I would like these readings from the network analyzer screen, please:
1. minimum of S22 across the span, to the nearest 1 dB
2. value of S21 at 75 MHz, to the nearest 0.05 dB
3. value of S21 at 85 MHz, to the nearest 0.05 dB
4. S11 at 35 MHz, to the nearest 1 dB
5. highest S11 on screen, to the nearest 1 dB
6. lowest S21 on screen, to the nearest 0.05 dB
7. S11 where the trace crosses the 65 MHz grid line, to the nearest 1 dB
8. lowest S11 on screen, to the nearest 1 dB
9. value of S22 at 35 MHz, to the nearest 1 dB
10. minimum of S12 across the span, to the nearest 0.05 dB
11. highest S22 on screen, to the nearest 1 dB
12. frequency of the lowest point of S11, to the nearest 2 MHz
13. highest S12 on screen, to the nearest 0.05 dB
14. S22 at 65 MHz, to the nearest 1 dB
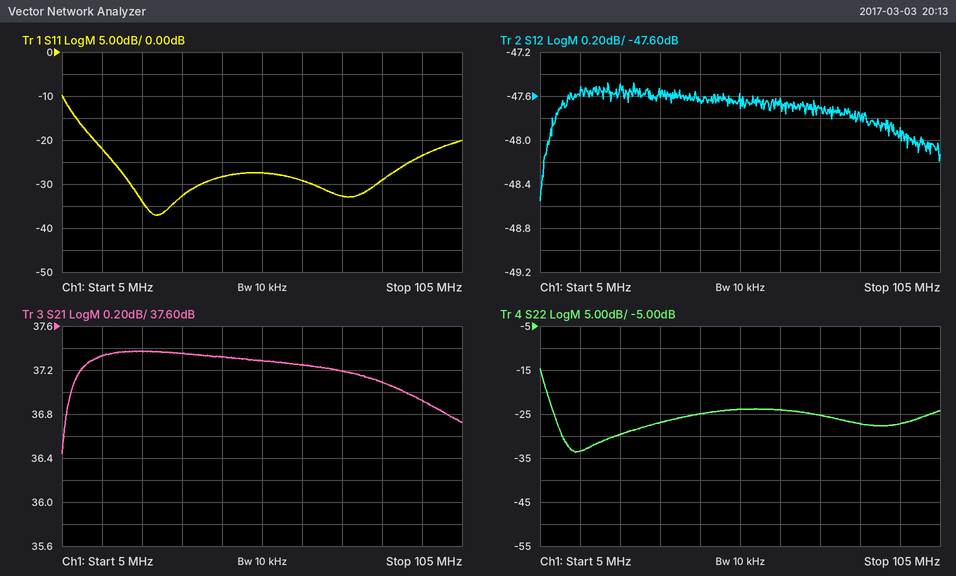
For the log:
-34 dB
37.20 dB
37.10 dB
-33 dB
-10 dB
36.45 dB
-29 dB
-37 dB
-27 dB
-48.55 dB
-15 dB
28 MHz
-47.50 dB
-24 dB
